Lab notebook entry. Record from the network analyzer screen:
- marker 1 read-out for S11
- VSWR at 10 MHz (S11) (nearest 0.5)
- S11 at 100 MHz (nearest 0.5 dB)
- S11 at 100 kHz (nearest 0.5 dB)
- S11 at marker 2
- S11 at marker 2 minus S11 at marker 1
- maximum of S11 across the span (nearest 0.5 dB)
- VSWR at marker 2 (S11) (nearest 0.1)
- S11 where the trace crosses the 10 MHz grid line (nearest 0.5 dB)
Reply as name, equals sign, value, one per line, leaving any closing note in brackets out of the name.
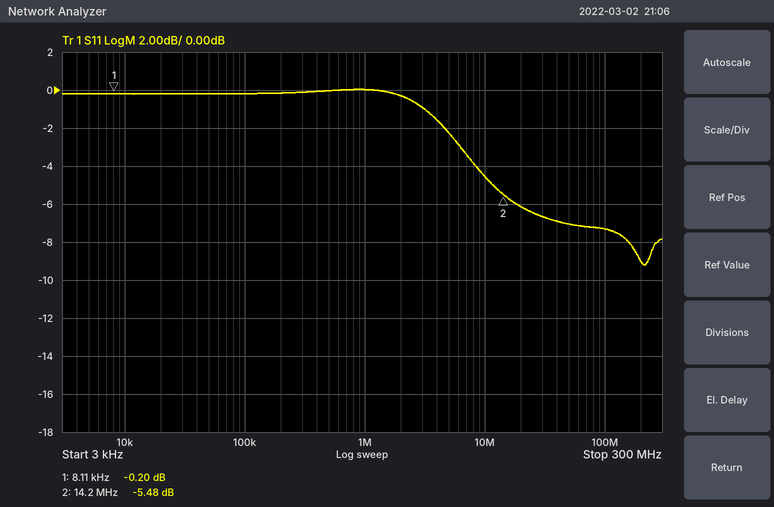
marker 1 read-out for S11 = -0.20 dB
VSWR at 10 MHz (S11) = 4.0
S11 at 100 MHz = -7.5 dB
S11 at 100 kHz = 0.0 dB
S11 at marker 2 = -5.48 dB
S11 at marker 2 minus S11 at marker 1 = -5.28 dB
maximum of S11 across the span = 0.0 dB
VSWR at marker 2 (S11) = 3.3
S11 where the trace crosses the 10 MHz grid line = -4.5 dB
